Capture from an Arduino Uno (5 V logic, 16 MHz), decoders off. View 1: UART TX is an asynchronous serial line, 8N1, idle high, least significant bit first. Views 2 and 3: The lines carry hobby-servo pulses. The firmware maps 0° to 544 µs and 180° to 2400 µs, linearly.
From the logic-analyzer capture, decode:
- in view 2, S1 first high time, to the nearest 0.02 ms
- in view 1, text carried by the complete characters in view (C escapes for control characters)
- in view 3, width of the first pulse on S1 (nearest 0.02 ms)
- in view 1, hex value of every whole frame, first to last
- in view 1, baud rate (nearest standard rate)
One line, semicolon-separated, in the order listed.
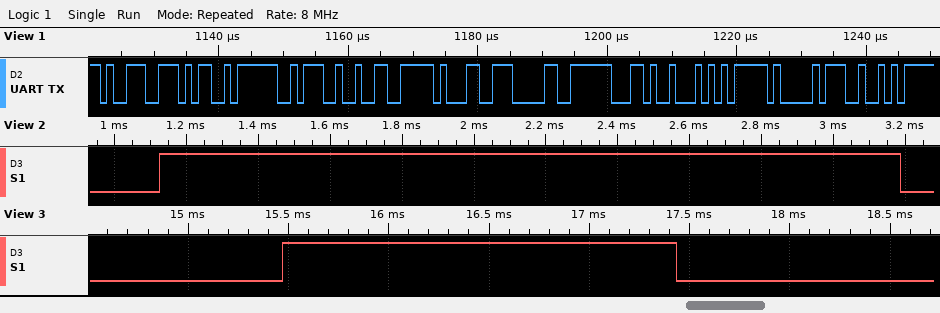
2.06 ms; "9M:210,TAR"; 1.96 ms; 0x39 0x4D 0x3A 0x32 0x31 0x30 0x2C 0x54 0x41 0x52; 1000000 baud
